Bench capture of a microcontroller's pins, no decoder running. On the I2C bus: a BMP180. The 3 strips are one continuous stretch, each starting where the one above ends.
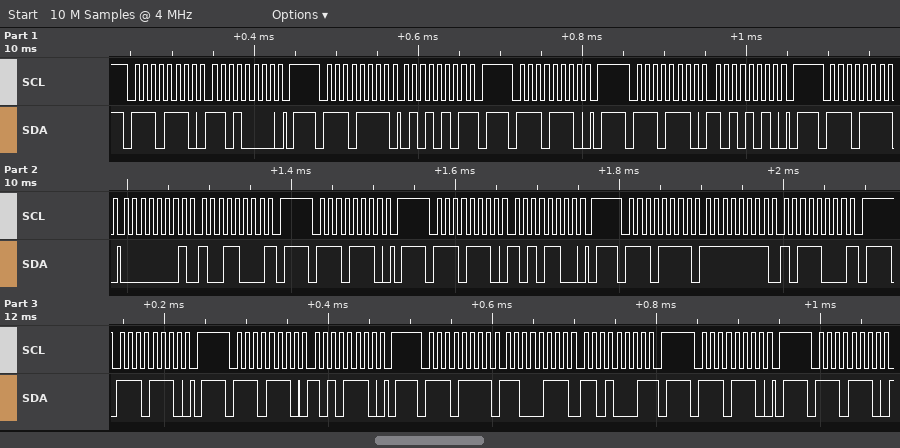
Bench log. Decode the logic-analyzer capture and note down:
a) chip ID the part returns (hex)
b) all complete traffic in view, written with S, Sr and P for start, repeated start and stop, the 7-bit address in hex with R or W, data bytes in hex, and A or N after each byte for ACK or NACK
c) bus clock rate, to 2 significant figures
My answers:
0x55
S 77W A D0 A P S 77R A 55 N P S 77W A P S 77W A AA A P S 77R A 01 A 98 N P S 77W A P S 77W A AC A P S 77R A FF A B8 N P S 77W A P S 77W A AE A P S 77R A C7 A D1 N P S 77W A P S 77W A
100 kHz
